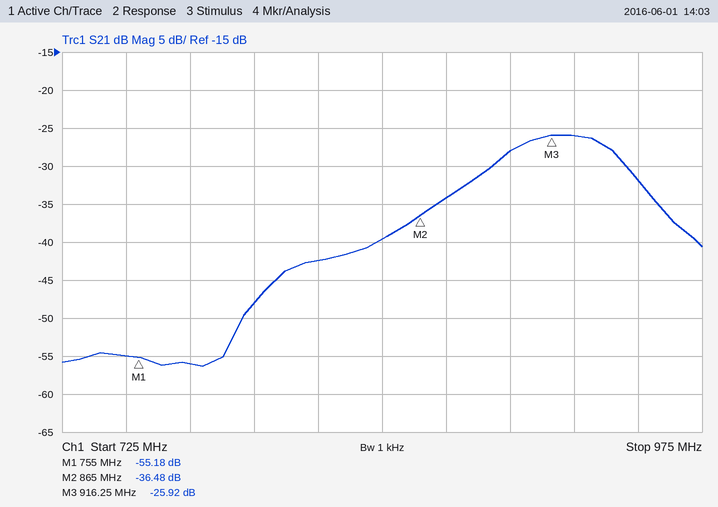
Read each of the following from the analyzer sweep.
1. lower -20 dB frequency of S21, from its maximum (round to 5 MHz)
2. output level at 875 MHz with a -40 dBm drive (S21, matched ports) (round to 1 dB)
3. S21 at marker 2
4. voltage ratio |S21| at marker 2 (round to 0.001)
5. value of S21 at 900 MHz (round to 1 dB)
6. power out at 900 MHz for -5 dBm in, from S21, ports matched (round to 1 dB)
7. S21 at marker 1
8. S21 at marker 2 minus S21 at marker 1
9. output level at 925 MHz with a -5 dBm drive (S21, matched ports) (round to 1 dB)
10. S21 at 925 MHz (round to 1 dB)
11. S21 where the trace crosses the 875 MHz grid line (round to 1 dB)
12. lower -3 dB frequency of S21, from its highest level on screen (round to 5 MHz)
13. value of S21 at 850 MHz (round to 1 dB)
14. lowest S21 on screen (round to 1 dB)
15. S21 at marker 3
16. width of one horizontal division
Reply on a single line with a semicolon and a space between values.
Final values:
805 MHz; -74 dBm; -36.48 dB; 0.015; -28 dB; -33 dBm; -55.18 dB; 18.70 dB; -31 dBm; -26 dB; -34 dB; 895 MHz; -40 dB; -56 dB; -25.92 dB; 25 MHz
